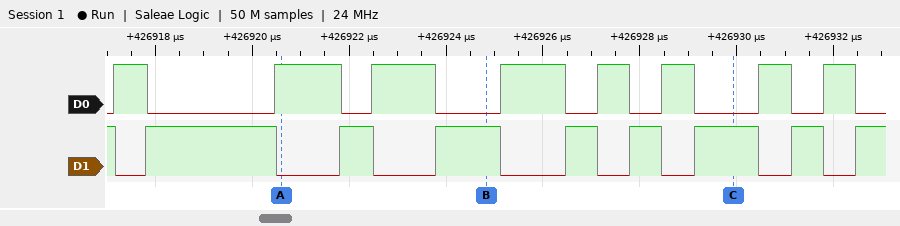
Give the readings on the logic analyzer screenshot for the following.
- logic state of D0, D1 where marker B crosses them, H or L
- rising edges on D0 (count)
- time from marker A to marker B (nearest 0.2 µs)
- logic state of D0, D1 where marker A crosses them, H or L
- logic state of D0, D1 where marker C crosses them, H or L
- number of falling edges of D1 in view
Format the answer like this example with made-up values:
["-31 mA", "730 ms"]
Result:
["D0=L, D1=H", "8", "4.2 µs", "D0=H, D1=L", "D0=L, D1=H", "8"]
